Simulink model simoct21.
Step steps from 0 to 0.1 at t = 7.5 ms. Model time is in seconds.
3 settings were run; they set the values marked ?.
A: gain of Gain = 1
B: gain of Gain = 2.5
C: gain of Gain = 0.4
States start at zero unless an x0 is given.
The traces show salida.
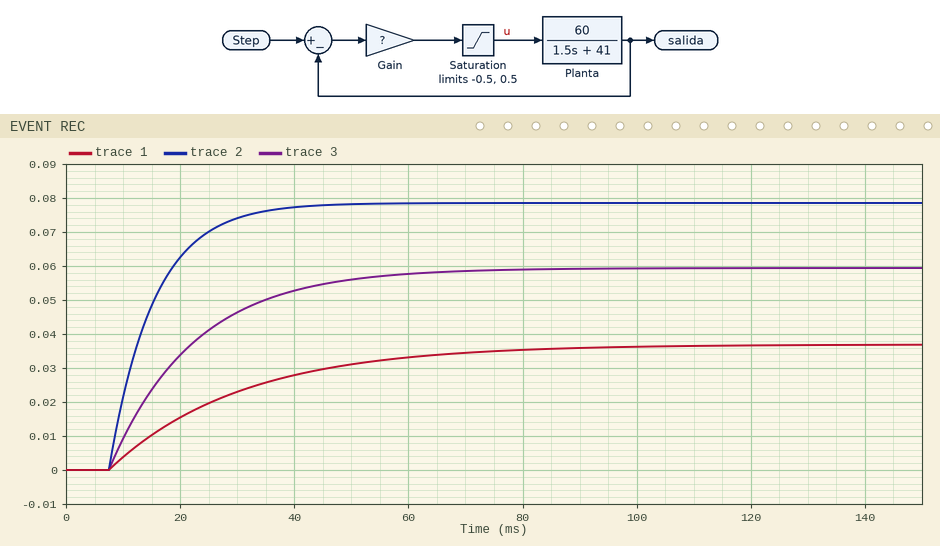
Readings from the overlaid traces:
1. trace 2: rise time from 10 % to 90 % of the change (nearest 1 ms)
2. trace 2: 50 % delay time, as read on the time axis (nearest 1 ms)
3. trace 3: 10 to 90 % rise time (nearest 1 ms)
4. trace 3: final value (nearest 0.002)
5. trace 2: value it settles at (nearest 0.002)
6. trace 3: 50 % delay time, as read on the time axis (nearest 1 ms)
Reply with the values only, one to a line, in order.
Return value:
17 ms
13 ms
33 ms
0.060
0.078
18 ms
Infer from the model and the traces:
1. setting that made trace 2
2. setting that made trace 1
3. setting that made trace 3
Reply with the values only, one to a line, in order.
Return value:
B
C
A
